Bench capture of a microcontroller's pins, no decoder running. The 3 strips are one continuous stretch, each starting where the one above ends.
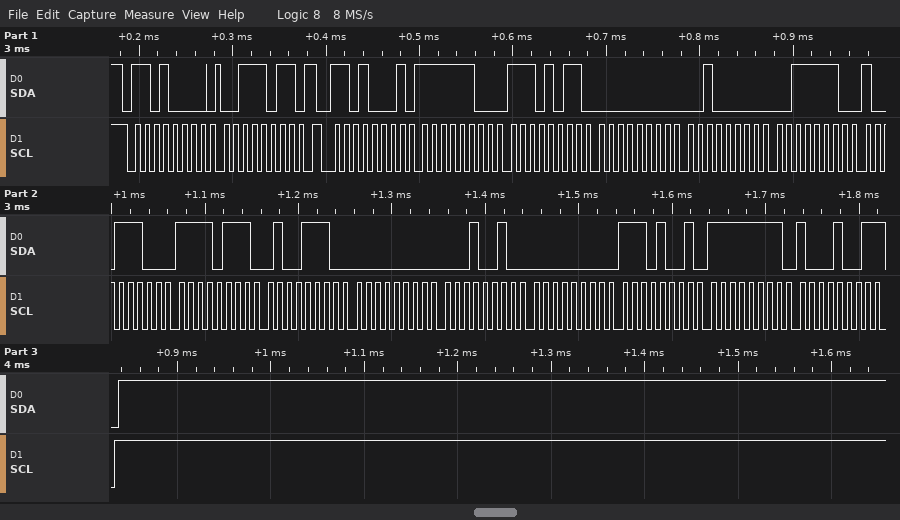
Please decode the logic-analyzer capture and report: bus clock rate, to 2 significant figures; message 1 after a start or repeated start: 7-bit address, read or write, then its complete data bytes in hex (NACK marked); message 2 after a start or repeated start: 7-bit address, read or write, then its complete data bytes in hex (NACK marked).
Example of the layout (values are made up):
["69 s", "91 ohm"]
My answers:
["100 kHz", "0x68 write: 3B", "0x68 read: FC EB 00 20 3E 9C F7 4E 00 12 00 E9 FF 89 NACK"]
